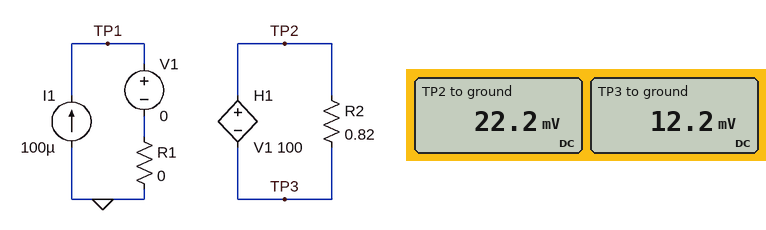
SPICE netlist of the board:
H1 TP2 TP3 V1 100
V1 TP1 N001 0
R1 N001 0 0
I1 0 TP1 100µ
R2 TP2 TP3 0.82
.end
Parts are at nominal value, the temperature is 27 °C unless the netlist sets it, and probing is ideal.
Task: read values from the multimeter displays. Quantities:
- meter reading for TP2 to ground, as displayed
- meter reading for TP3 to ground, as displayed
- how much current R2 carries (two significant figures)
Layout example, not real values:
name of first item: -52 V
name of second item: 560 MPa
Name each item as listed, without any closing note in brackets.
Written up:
meter reading for TP2 to ground, as displayed: 22.2 mV
meter reading for TP3 to ground, as displayed: 12.2 mV
how much current R2 carries: 12 mA
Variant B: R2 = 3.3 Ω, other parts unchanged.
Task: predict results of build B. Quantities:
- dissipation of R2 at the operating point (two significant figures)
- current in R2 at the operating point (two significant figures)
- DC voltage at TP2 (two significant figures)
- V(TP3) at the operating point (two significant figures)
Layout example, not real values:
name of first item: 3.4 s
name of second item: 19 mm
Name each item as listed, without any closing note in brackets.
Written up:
dissipation of R2 at the operating point: 30 µW
current in R2 at the operating point: 3.0 mA
DC voltage at TP2: 13 mV
V(TP3) at the operating point: 3.0 mV
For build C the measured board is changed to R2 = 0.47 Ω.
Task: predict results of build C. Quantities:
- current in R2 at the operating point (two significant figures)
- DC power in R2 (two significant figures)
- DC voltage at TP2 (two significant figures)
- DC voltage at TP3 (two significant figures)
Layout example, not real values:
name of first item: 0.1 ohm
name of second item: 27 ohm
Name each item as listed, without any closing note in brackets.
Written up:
current in R2 at the operating point: 21 mA
DC power in R2: 210 µW
DC voltage at TP2: 31 mV
DC voltage at TP3: 21 mV
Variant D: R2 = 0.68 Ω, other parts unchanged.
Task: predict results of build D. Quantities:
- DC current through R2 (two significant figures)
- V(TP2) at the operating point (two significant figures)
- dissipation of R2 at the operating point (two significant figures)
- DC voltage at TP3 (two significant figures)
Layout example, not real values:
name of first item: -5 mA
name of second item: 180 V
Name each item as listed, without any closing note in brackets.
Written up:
DC current through R2: 15 mA
V(TP2) at the operating point: 25 mV
dissipation of R2 at the operating point: 150 µW
DC voltage at TP3: 15 mV
